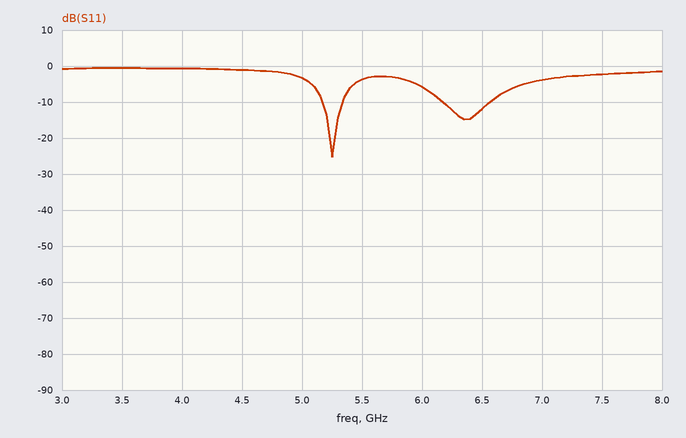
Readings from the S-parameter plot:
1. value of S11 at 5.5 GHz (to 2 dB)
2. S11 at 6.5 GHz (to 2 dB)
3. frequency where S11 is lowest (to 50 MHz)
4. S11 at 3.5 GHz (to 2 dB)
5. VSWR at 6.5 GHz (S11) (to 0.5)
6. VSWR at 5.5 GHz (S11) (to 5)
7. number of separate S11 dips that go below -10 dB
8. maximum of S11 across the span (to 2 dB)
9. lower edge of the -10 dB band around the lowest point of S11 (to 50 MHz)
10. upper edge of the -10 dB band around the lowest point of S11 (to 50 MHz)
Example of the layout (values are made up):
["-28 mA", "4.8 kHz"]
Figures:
["-4 dB", "-12 dB", "5.25 GHz", "0 dB", "1.5", "5", "2", "0 dB", "5.15 GHz", "5.35 GHz"]
